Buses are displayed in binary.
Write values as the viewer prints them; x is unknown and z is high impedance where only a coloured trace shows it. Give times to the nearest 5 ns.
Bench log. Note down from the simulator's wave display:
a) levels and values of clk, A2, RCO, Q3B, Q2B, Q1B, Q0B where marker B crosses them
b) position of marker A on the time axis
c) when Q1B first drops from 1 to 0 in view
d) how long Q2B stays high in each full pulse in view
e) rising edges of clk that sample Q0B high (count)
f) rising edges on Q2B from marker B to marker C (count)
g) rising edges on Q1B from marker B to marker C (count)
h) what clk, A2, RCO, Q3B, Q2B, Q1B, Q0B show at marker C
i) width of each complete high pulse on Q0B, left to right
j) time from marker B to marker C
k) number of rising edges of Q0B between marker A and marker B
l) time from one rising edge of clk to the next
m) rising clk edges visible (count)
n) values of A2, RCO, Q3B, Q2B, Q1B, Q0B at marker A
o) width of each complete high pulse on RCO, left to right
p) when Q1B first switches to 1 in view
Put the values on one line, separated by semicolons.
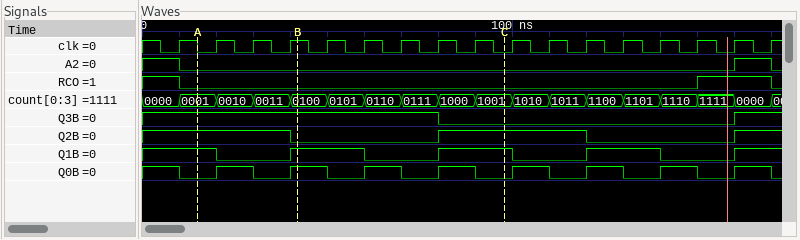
clk=1, A2=0, RCO=0, Q3B=1, Q2B=0, Q1B=1, Q0B=1; 15 ns; 20 ns; 40 ns; 9; 1; 1; clk=0, A2=0, RCO=0, Q3B=0, Q2B=1, Q1B=1, Q0B=0; 10 ns, 10 ns, 10 ns, 10 ns, 10 ns, 10 ns, 10 ns, 10 ns; 55 ns; 2; 10 ns; 17; A2=0, RCO=0, Q3B=1, Q2B=1, Q1B=1, Q0B=0; 20 ns; 40 ns
